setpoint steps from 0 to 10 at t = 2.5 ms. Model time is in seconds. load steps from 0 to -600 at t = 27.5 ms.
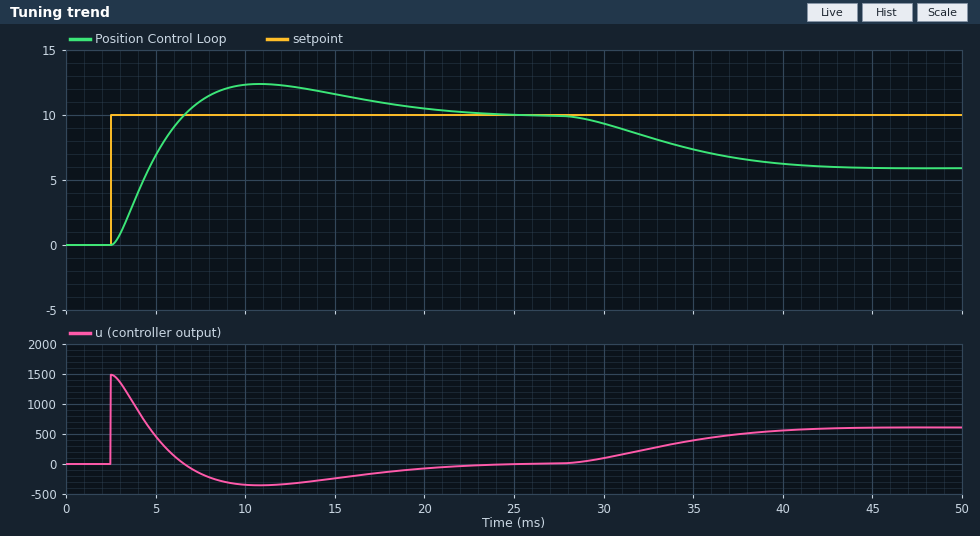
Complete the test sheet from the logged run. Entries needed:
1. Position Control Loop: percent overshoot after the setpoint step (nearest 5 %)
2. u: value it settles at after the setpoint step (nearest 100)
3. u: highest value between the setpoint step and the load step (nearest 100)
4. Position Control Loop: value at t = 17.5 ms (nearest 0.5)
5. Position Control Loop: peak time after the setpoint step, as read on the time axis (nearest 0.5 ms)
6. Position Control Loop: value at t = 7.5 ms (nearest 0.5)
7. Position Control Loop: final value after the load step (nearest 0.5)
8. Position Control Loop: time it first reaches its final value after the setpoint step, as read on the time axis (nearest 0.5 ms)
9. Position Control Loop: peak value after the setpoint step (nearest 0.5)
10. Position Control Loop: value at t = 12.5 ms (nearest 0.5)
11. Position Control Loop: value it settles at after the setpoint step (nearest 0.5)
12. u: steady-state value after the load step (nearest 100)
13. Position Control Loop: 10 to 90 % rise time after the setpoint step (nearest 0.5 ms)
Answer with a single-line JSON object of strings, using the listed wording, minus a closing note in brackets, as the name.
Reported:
{"Position Control Loop: percent overshoot after the setpoint step": "25 %", "u: value it settles at after the setpoint step": "0", "u: highest value between the setpoint step and the load step": "1500", "Position Control Loop: value at t = 17.5 ms": "11.0", "Position Control Loop: peak time after the setpoint step, as read on the time axis": "11.0 ms", "Position Control Loop: value at t = 7.5 ms": "11.0", "Position Control Loop: final value after the load step": "6.0", "Position Control Loop: time it first reaches its final value after the setpoint step, as read on the time axis": "6.5 ms", "Position Control Loop: peak value after the setpoint step": "12.5", "Position Control Loop: value at t = 12.5 ms": "12.0", "Position Control Loop: value it settles at after the setpoint step": "10.0", "u: steady-state value after the load step": "600", "Position Control Loop: 10 to 90 % rise time after the setpoint step": "3.0 ms"}
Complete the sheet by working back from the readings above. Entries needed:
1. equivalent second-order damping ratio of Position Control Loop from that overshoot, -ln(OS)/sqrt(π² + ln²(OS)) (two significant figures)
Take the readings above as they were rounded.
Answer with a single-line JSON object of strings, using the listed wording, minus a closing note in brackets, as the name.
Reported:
{"equivalent second-order damping ratio of Position Control Loop from that overshoot, -ln(OS)/sqrt(π² + ln²(OS))": "0.40"}
